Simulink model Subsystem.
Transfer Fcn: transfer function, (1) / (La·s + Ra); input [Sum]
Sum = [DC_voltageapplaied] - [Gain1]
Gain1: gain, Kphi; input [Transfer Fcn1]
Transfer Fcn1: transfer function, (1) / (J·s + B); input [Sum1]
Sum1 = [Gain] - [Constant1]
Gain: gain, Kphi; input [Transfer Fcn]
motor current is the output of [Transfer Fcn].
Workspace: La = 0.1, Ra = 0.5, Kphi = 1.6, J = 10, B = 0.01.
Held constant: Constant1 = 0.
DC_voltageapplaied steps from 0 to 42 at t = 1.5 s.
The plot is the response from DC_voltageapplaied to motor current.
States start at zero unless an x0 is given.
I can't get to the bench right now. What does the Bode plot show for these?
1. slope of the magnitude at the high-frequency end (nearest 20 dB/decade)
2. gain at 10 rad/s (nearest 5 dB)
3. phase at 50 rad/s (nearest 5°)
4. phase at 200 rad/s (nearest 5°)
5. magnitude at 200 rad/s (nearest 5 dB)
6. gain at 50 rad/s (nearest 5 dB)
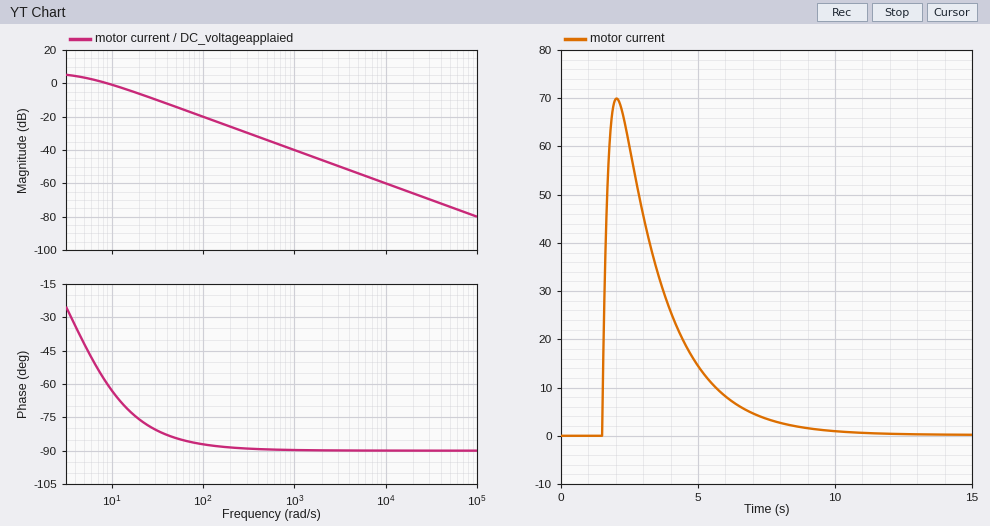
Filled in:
-20 dB/decade
0 dB
-85°
-90°
-25 dB
-15 dB
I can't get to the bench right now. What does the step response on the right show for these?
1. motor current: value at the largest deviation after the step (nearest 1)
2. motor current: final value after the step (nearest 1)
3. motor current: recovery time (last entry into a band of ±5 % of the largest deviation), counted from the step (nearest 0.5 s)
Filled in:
70
0
6.0 s
